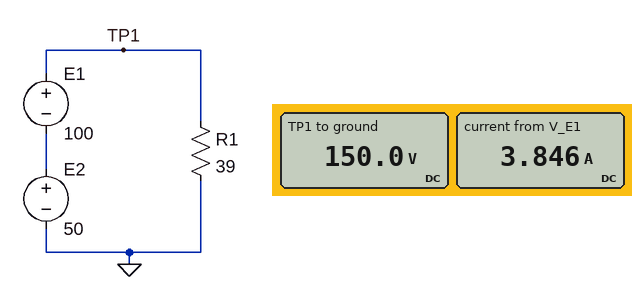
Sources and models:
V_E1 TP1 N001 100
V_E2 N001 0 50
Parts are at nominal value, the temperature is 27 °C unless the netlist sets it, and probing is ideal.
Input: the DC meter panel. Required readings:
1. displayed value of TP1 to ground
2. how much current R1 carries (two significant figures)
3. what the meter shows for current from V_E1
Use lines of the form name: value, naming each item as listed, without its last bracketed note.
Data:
displayed value of TP1 to ground: 150.0 V
how much current R1 carries: 3.8 A
what the meter shows for current from V_E1: 3.846 A
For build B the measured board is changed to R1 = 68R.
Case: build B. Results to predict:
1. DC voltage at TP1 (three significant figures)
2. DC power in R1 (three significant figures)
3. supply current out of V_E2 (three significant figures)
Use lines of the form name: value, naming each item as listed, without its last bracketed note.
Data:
DC voltage at TP1: 150 V
DC power in R1: 331 W
supply current out of V_E2: 2.21 A
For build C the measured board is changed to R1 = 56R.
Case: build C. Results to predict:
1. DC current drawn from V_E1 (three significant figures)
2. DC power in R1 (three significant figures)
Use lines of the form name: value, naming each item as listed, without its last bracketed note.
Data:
DC current drawn from V_E1: 2.68 A
DC power in R1: 402 W
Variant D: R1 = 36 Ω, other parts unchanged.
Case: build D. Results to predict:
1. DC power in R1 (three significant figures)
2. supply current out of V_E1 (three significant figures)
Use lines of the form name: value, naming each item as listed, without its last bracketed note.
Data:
DC power in R1: 625 W
supply current out of V_E1: 4.17 A
